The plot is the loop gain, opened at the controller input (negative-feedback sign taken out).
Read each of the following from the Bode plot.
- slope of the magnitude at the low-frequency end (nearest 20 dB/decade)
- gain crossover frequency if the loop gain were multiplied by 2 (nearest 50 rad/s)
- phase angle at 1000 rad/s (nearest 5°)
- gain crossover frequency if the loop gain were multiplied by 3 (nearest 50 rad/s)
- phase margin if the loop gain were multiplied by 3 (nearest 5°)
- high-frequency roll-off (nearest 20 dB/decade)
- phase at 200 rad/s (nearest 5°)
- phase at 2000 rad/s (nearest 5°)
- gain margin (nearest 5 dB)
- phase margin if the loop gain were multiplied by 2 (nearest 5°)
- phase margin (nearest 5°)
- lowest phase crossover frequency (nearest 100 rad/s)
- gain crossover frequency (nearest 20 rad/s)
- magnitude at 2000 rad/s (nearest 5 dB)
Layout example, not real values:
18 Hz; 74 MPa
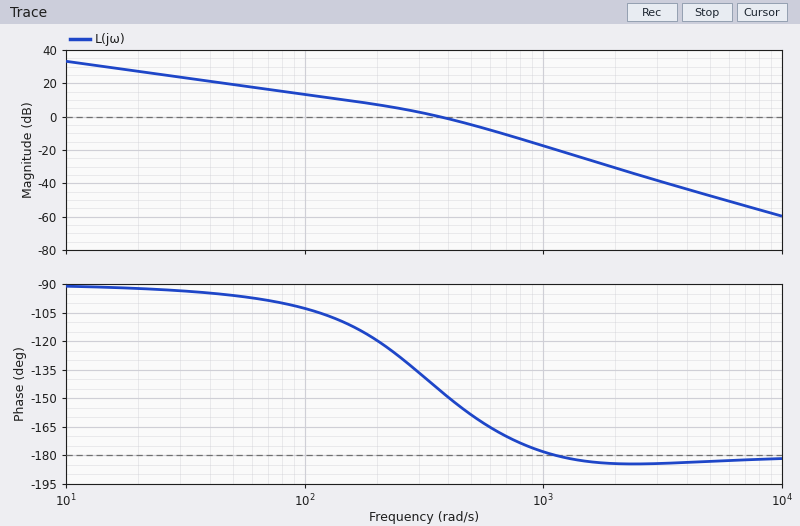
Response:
-20 dB/decade; 550 rad/s; -180°; 650 rad/s; 10°; -40 dB/decade; -120°; -185°; 20 dB; 20°; 35°; 1100 rad/s; 360 rad/s; -30 dB
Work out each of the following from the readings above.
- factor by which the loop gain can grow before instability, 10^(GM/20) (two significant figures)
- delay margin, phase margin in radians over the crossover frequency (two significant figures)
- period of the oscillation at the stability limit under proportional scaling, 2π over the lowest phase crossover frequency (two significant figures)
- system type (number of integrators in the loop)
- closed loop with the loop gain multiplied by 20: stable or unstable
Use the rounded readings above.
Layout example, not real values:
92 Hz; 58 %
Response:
10; 0.0017 s; 0.0057 s; 1; unstable
